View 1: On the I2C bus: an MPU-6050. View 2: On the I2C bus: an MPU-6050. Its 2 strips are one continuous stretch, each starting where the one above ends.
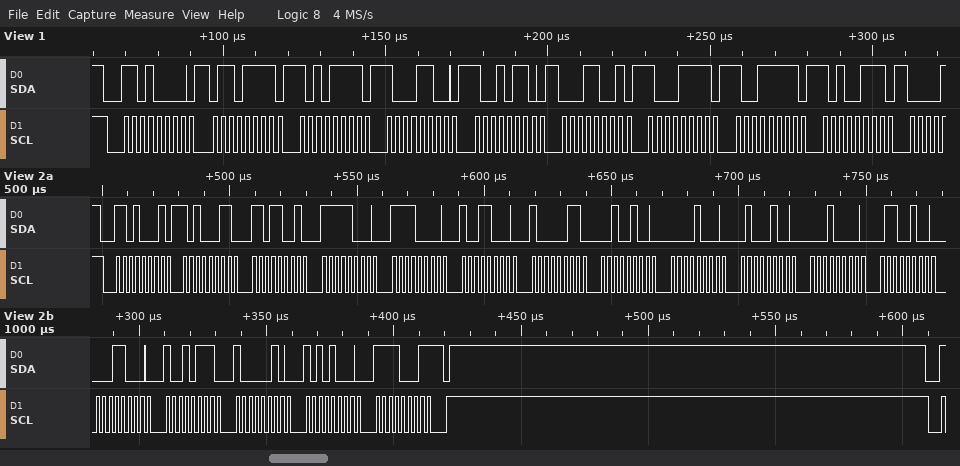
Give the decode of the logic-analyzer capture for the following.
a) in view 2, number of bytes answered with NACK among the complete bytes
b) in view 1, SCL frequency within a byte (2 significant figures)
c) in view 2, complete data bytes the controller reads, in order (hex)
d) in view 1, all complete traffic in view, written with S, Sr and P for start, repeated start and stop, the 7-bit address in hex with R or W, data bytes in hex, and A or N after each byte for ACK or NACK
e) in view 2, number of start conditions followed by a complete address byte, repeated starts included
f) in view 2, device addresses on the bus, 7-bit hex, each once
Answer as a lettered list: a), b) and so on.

a) 1
b) 400 kHz
c) A3 D9 F8 F0 98 83 24 08 44 10 64 18 97 82 A8 F1
d) S 68W A 6F A AF A 8C A 96 A 19 A 8F A 9F A A7 A
e) 1
f) 0x68
